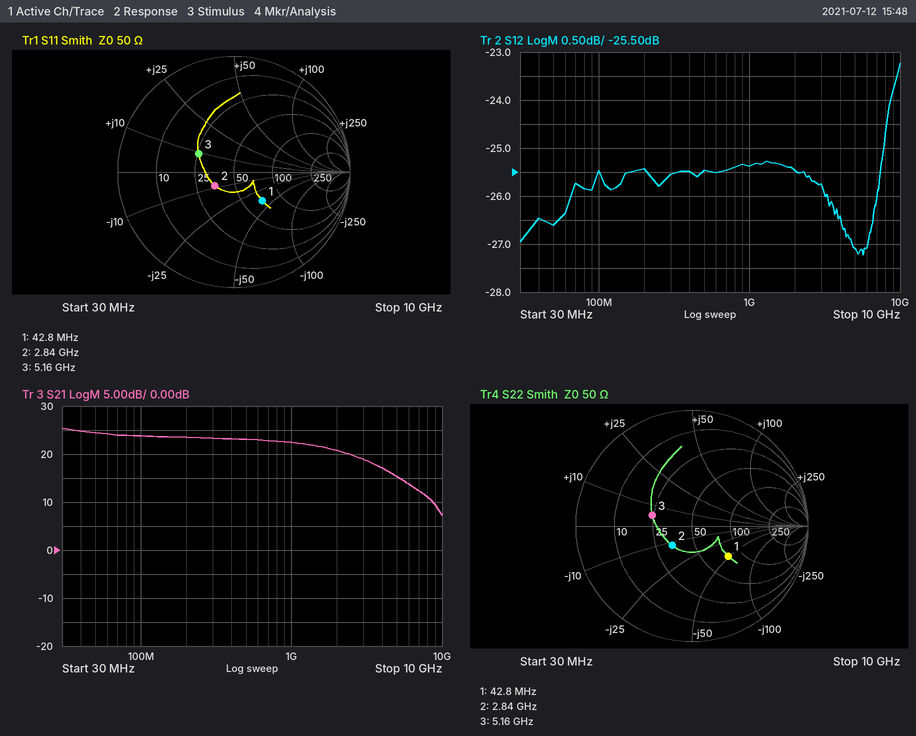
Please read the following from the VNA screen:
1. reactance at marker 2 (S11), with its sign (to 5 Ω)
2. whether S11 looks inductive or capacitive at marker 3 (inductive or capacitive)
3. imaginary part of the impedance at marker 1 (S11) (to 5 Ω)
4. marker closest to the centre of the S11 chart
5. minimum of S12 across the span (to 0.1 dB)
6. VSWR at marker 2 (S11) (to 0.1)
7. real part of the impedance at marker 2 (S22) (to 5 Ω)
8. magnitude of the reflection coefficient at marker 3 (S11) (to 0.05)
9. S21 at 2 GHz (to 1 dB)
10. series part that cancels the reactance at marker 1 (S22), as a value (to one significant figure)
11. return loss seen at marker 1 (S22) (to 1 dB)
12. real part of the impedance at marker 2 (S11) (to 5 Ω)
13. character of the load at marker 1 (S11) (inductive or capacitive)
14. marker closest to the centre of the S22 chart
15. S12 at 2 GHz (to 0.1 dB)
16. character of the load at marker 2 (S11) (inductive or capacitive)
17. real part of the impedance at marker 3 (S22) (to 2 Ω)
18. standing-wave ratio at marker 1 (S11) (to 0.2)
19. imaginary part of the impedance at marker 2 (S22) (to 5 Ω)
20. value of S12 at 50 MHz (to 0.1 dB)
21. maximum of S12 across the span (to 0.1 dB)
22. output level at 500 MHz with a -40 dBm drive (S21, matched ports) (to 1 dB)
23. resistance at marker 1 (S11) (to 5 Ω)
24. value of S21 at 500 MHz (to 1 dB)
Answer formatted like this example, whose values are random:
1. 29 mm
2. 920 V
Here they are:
1. -10 Ω
2. inductive
3. -40 Ω
4. marker 2
5. -27.2 dB
6. 1.5
7. 35 Ω
8. 0.35
9. 21 dB
10. 200 nH
11. 8 dB
12. 35 Ω
13. capacitive
14. marker 2
15. -25.5 dB
16. capacitive
17. 24 Ω
18. 2.0
19. -10 Ω
20. -26.6 dB
21. -23.2 dB
22. -17 dBm
23. 70 Ω
24. 23 dB
